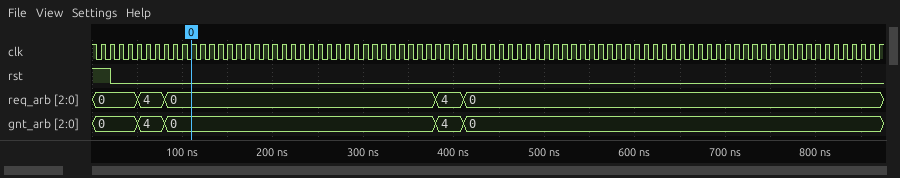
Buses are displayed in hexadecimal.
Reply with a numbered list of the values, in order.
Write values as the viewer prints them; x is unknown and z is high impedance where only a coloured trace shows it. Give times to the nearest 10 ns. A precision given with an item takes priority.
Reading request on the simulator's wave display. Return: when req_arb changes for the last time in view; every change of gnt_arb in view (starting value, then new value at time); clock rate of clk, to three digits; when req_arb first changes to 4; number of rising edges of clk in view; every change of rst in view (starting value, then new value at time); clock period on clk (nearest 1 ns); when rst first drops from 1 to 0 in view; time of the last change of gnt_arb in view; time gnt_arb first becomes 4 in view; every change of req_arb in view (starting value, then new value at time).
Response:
1. 410 ns
2. 0, 4 at 50 ns, 0 at 80 ns, 4 at 380 ns, 0 at 410 ns
3. 100 MHz
4. 50 ns
5. 87
6. 1, 0 at 20 ns
7. 10 ns
8. 20 ns
9. 410 ns
10. 50 ns
11. 0, 4 at 50 ns, 0 at 80 ns, 4 at 380 ns, 0 at 410 ns
